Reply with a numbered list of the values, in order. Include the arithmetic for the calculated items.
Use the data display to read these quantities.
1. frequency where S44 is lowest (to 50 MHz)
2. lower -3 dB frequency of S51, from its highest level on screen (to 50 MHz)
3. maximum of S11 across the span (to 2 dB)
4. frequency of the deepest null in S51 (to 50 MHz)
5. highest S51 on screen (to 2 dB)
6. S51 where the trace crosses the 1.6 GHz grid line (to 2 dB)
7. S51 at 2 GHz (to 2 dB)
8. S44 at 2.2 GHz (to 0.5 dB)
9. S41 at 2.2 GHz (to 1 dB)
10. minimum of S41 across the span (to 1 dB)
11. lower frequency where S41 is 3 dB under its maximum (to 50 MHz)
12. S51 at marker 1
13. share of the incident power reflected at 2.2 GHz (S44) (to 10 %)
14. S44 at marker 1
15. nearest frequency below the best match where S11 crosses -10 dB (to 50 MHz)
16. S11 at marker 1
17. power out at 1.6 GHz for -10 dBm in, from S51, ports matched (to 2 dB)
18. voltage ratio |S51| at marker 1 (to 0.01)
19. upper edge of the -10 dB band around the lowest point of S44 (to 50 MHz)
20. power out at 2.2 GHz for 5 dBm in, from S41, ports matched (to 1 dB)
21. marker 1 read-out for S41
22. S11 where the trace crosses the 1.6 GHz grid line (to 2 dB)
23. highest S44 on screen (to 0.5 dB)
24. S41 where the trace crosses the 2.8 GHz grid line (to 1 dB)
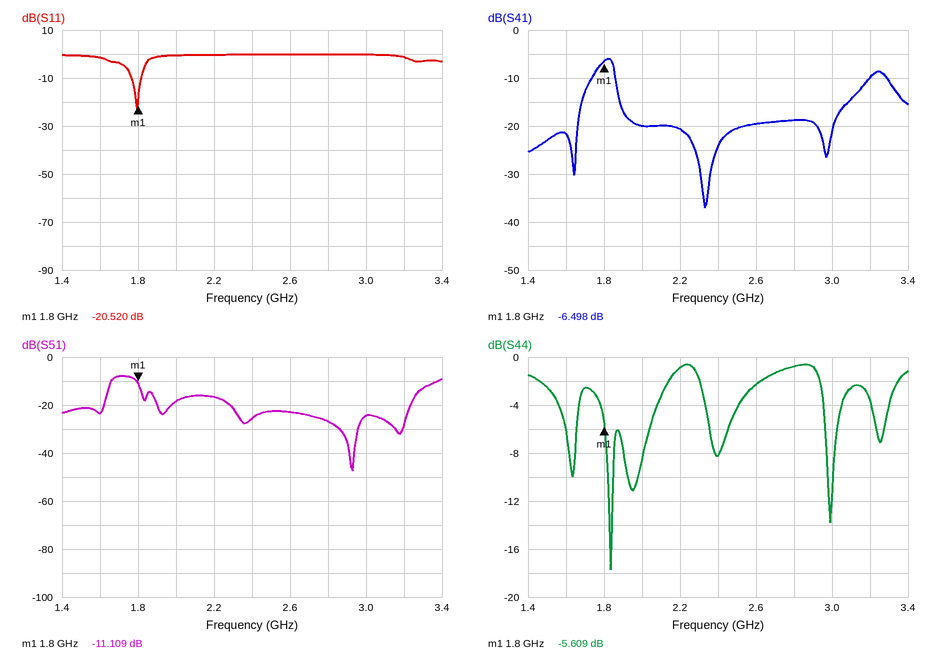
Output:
1. 1.85 GHz
2. 1.65 GHz
3. 0 dB
4. 2.95 GHz
5. -8 dB
6. -24 dB
7. -18 dB
8. -1.0 dB
9. -21 dB
10. -37 dB
11. 1.75 GHz
12. -11.109 dB
13. 10^(-1/10) ≈ 79.4 %, so 80 % to the nearest 10 %
14. -5.609 dB
15. 1.75 GHz
16. -20.520 dB
17. -10 dBm + (-24 dB) = -34 dBm
18. 10^(-11.109/20) ≈ 0.28
19. 1.85 GHz
20. 5 dBm + (-21 dB) = -16 dBm
21. -6.498 dB
22. -2 dB
23. -0.5 dB
24. -19 dB
